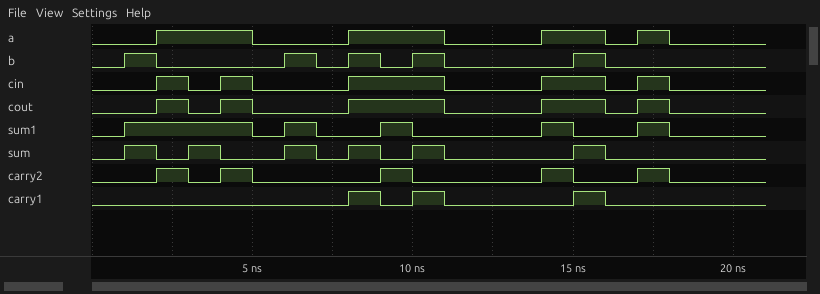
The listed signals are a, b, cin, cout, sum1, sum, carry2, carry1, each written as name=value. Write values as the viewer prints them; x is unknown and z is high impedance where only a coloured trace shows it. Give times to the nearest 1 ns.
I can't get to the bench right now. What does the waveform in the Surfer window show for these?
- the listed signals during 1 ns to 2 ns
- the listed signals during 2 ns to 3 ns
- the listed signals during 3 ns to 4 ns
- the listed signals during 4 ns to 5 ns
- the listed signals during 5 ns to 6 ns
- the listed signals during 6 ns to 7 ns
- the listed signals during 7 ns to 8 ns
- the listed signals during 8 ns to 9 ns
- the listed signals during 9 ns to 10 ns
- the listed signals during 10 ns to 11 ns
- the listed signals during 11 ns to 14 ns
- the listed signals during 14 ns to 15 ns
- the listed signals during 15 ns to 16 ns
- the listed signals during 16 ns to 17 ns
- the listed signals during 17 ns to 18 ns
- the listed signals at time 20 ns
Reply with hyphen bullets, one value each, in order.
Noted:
- a=0, b=1, cin=0, cout=0, sum1=1, sum=1, carry2=0, carry1=0
- a=1, b=0, cin=1, cout=1, sum1=1, sum=0, carry2=1, carry1=0
- a=1, b=0, cin=0, cout=0, sum1=1, sum=1, carry2=0, carry1=0
- a=1, b=0, cin=1, cout=1, sum1=1, sum=0, carry2=1, carry1=0
- a=0, b=0, cin=0, cout=0, sum1=0, sum=0, carry2=0, carry1=0
- a=0, b=1, cin=0, cout=0, sum1=1, sum=1, carry2=0, carry1=0
- a=0, b=0, cin=0, cout=0, sum1=0, sum=0, carry2=0, carry1=0
- a=1, b=1, cin=1, cout=1, sum1=0, sum=1, carry2=0, carry1=1
- a=1, b=0, cin=1, cout=1, sum1=1, sum=0, carry2=1, carry1=0
- a=1, b=1, cin=1, cout=1, sum1=0, sum=1, carry2=0, carry1=1
- a=0, b=0, cin=0, cout=0, sum1=0, sum=0, carry2=0, carry1=0
- a=1, b=0, cin=1, cout=1, sum1=1, sum=0, carry2=1, carry1=0
- a=1, b=1, cin=1, cout=1, sum1=0, sum=1, carry2=0, carry1=1
- a=0, b=0, cin=0, cout=0, sum1=0, sum=0, carry2=0, carry1=0
- a=1, b=0, cin=1, cout=1, sum1=1, sum=0, carry2=1, carry1=0
- a=0, b=0, cin=0, cout=0, sum1=0, sum=0, carry2=0, carry1=0
